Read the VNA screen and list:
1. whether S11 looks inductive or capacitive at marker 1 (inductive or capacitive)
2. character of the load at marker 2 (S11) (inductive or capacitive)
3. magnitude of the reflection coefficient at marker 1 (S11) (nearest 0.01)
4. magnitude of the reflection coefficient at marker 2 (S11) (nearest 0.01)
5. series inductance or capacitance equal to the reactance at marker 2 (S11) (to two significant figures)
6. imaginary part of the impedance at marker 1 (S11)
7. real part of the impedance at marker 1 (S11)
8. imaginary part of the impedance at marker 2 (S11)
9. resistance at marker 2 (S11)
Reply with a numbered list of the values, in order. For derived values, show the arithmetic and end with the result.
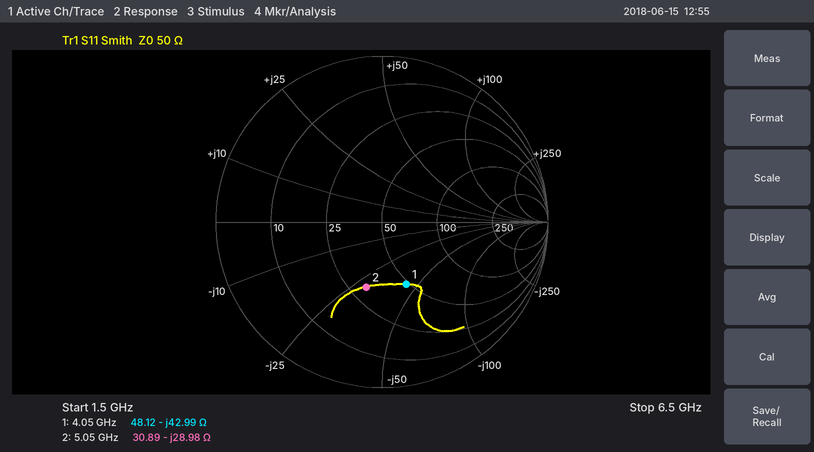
1. capacitive
2. capacitive
3. 0.40
4. 0.40
5. C = 1/(2π × 5.05 GHz × 28.98 Ω) ≈ 1.1 pF
6. -42.99 Ω
7. 48.12 Ω
8. -28.98 Ω
9. 30.89 Ω
